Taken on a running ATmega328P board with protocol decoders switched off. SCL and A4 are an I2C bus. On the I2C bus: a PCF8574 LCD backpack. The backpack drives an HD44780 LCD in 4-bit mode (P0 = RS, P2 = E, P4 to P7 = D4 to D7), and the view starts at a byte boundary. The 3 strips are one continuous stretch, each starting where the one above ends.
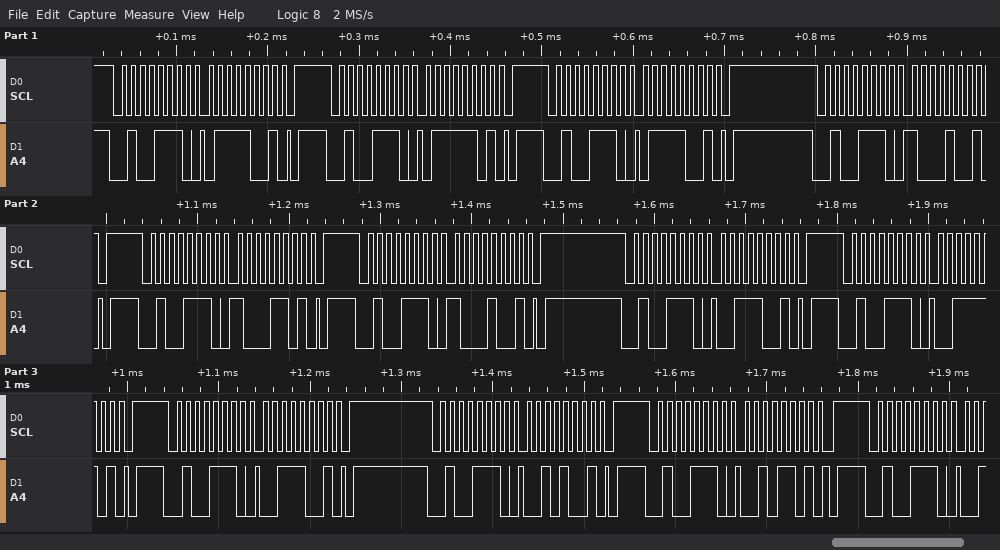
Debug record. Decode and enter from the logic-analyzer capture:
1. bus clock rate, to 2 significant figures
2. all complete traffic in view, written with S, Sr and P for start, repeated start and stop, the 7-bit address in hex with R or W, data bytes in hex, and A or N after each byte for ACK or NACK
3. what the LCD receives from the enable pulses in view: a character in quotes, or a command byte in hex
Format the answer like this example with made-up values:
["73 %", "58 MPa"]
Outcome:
["100 kHz", "S 27W A 79 A P S 27W A 7D A P S 27W A 79 A P S 27W A 89 A P S 27W A 8D A P S 27W A 89 A P S 27W A 39 A P S 27W A 3D A P S 27W A 39 A P S 27W A 29 A P S 27W A 2D A P S 27W A", "'x'"]
